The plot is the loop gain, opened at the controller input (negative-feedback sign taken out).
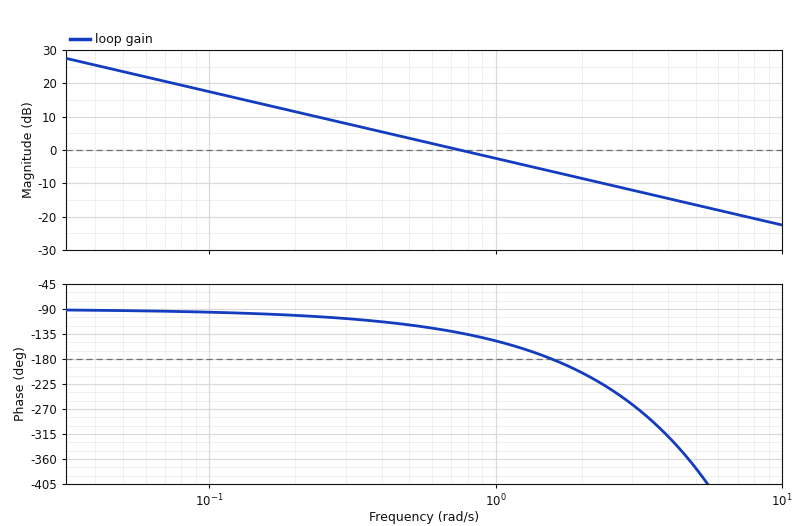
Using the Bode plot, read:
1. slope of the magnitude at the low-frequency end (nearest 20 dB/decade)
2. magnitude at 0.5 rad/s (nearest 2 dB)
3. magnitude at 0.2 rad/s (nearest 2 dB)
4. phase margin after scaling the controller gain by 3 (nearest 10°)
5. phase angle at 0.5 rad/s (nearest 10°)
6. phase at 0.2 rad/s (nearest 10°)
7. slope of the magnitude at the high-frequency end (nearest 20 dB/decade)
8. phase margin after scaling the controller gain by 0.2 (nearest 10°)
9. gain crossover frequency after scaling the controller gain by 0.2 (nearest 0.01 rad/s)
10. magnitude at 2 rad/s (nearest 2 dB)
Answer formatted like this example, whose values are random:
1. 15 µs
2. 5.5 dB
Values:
1. -20 dB/decade
2. 4 dB
3. 12 dB
4. -40°
5. -120°
6. -100°
7. -20 dB/decade
8. 80°
9. 0.15 rad/s
10. -8 dB
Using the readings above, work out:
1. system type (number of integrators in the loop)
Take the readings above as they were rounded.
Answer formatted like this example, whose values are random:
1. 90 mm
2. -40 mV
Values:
1. 1
